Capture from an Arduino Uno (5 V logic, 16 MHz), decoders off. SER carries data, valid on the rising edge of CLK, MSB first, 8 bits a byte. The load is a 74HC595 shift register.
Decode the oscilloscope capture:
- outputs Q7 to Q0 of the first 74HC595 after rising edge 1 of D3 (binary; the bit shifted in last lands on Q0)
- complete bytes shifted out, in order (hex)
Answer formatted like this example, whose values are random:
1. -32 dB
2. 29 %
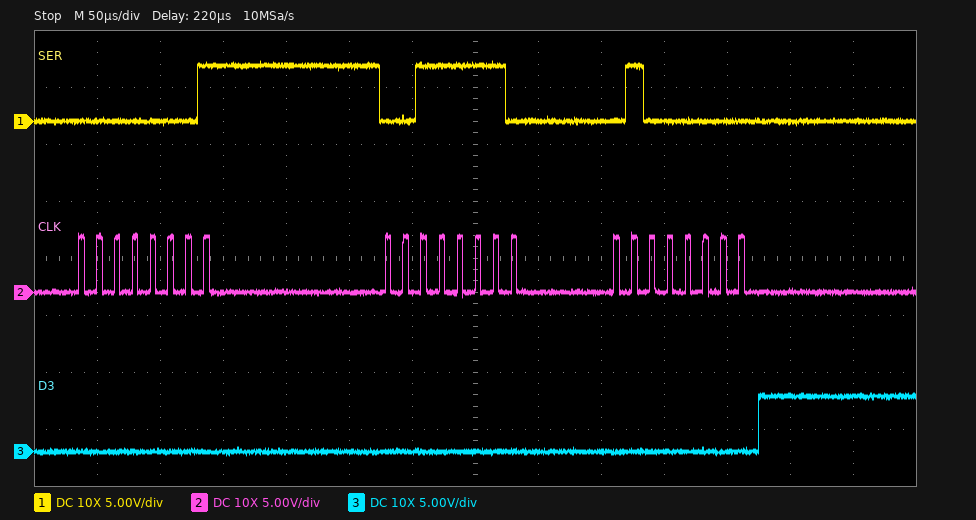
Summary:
1. 01000000
2. 0x01 0x3E 0x40
